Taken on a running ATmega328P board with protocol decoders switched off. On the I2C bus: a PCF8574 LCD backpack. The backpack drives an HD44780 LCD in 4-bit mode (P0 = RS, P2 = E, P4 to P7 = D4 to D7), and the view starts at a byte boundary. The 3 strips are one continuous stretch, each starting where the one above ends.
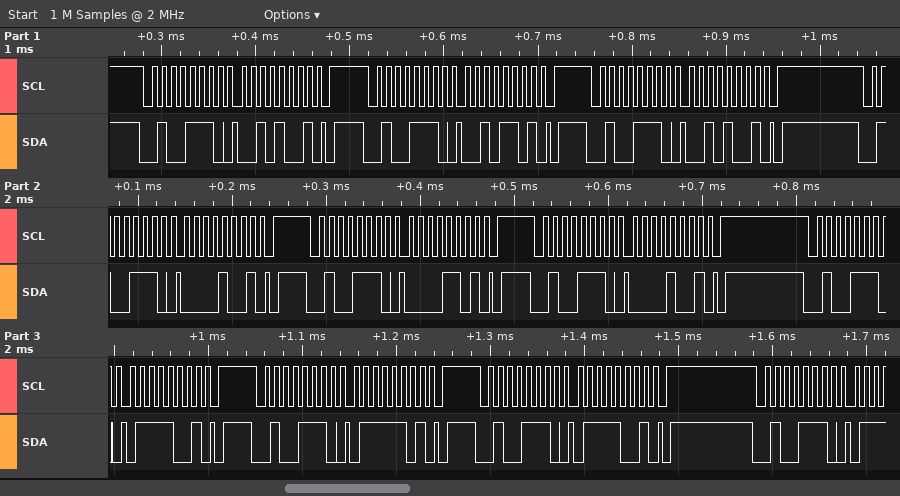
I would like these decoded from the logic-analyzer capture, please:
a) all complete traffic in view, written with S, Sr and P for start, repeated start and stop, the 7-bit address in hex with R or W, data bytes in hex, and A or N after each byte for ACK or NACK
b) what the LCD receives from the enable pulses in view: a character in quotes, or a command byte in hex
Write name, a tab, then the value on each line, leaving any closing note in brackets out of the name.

all complete traffic in view, written with S, Sr and P for start, repeated start and stop, the 7-bit address in hex with R or W, data bytes in hex, and A or N after each byte for ACK or NACK	S 27W A 29 A P S 27W A 2D A P S 27W A 29 A P S 27W A 09 A P S 27W A 0D A P S 27W A 09 A P S 27W A 79 A P S 27W A 7D A P S 27W A 79 A P S 27W A
what the LCD receives from the enable pulses in view: a character in quotes, or a command byte in hex	' '
